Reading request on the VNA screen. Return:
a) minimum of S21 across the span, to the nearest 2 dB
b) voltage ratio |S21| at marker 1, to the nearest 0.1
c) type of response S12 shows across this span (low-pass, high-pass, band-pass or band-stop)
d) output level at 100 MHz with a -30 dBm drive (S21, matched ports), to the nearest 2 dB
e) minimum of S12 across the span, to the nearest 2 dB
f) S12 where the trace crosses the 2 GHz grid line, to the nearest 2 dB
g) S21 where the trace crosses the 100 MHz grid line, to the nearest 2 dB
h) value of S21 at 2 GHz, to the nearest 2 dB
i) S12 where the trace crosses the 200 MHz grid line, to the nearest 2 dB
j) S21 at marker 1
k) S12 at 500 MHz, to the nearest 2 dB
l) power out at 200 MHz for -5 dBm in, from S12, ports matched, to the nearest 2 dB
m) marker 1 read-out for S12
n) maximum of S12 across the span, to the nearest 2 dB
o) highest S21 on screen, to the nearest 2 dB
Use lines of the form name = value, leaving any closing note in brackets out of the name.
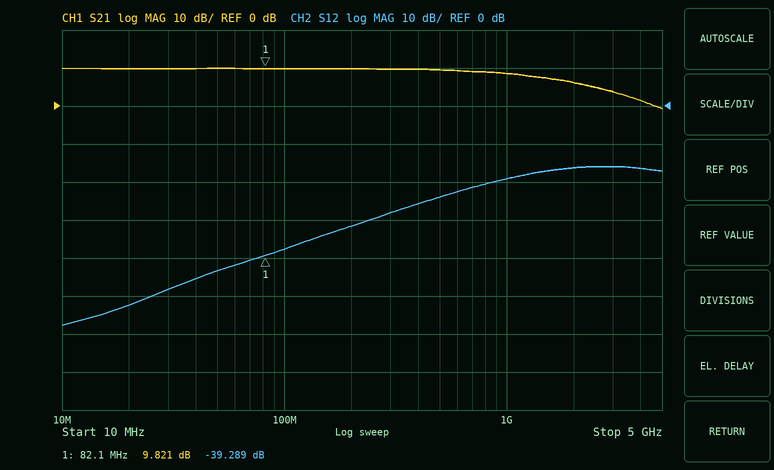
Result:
minimum of S21 across the span, to the nearest 2 dB = 0 dB
voltage ratio |S21| at marker 1, to the nearest 0.1 = 3.1
type of response S12 shows across this span = high-pass
output level at 100 MHz with a -30 dBm drive (S21, matched ports), to the nearest 2 dB = -20 dBm
minimum of S12 across the span, to the nearest 2 dB = -58 dB
S12 where the trace crosses the 2 GHz grid line, to the nearest 2 dB = -16 dB
S21 where the trace crosses the 100 MHz grid line, to the nearest 2 dB = 10 dB
value of S21 at 2 GHz, to the nearest 2 dB = 6 dB
S12 where the trace crosses the 200 MHz grid line, to the nearest 2 dB = -32 dB
S21 at marker 1 = 9.821 dB
S12 at 500 MHz, to the nearest 2 dB = -24 dB
power out at 200 MHz for -5 dBm in, from S12, ports matched, to the nearest 2 dB = -36 dBm
marker 1 read-out for S12 = -39.289 dB
maximum of S12 across the span, to the nearest 2 dB = -16 dB
highest S21 on screen, to the nearest 2 dB = 10 dB
